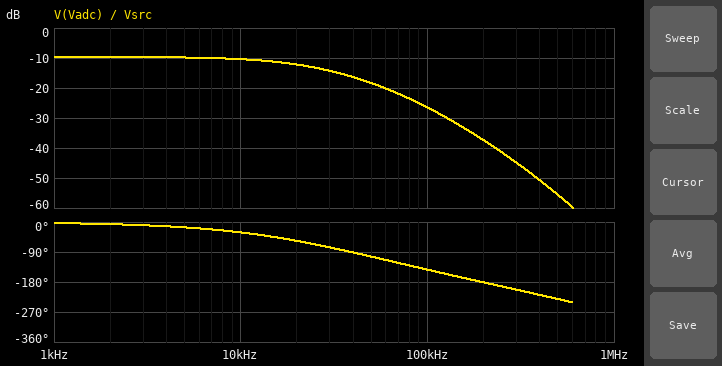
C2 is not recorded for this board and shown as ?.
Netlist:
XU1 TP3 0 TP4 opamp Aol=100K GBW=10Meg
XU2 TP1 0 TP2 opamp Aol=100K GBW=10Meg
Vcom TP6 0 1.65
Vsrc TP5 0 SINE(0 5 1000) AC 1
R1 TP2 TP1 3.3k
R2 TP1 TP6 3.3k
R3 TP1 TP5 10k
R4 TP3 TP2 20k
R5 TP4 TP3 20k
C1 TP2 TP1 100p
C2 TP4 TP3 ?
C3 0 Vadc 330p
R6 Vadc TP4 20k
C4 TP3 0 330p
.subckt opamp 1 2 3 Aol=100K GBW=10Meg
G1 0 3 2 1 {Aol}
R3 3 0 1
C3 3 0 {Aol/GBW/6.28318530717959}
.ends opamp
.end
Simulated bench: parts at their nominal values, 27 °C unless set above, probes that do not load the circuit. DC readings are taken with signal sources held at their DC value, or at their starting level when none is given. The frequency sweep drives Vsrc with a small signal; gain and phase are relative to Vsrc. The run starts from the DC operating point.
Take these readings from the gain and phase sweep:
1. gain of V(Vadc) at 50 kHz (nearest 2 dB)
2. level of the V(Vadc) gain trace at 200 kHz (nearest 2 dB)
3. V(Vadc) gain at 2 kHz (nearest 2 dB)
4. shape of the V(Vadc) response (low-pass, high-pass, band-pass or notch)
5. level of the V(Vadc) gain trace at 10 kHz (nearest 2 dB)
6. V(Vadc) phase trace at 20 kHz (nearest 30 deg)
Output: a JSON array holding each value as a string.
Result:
["-18 dB", "-38 dB", "-10 dB", "low-pass", "-10 dB", "-60 deg"]
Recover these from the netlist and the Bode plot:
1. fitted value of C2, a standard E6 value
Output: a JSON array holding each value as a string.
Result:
["100 pF"]
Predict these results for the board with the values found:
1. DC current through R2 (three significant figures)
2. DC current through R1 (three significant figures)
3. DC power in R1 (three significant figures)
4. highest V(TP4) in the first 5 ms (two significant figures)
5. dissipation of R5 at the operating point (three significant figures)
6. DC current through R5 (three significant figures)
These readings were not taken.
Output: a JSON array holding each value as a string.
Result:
["500 µA", "500 µA", "825 µW", "3.3 V", "136 µW", "82.5 µA"]
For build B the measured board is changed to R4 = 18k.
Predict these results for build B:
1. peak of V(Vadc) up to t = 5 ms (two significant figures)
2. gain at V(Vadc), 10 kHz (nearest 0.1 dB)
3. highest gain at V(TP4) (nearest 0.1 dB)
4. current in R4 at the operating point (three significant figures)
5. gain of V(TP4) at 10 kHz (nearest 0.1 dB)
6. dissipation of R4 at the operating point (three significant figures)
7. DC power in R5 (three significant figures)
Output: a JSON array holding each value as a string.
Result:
["3.7 V", "-9.5 dB", "-8.7 dB", "91.7 µA", "-8.8 dB", "151 µW", "168 µW"]
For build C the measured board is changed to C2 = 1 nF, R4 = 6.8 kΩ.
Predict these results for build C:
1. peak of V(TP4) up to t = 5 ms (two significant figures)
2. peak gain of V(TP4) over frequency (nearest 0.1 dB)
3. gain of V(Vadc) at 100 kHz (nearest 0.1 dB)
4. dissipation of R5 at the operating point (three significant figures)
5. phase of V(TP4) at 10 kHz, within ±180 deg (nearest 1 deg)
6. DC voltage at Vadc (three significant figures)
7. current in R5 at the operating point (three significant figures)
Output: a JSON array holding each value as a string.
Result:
["9.7 V", "-0.3 dB", "-35.1 dB", "1.18 mW", "-53 deg", "4.85 V", "243 µA"]
